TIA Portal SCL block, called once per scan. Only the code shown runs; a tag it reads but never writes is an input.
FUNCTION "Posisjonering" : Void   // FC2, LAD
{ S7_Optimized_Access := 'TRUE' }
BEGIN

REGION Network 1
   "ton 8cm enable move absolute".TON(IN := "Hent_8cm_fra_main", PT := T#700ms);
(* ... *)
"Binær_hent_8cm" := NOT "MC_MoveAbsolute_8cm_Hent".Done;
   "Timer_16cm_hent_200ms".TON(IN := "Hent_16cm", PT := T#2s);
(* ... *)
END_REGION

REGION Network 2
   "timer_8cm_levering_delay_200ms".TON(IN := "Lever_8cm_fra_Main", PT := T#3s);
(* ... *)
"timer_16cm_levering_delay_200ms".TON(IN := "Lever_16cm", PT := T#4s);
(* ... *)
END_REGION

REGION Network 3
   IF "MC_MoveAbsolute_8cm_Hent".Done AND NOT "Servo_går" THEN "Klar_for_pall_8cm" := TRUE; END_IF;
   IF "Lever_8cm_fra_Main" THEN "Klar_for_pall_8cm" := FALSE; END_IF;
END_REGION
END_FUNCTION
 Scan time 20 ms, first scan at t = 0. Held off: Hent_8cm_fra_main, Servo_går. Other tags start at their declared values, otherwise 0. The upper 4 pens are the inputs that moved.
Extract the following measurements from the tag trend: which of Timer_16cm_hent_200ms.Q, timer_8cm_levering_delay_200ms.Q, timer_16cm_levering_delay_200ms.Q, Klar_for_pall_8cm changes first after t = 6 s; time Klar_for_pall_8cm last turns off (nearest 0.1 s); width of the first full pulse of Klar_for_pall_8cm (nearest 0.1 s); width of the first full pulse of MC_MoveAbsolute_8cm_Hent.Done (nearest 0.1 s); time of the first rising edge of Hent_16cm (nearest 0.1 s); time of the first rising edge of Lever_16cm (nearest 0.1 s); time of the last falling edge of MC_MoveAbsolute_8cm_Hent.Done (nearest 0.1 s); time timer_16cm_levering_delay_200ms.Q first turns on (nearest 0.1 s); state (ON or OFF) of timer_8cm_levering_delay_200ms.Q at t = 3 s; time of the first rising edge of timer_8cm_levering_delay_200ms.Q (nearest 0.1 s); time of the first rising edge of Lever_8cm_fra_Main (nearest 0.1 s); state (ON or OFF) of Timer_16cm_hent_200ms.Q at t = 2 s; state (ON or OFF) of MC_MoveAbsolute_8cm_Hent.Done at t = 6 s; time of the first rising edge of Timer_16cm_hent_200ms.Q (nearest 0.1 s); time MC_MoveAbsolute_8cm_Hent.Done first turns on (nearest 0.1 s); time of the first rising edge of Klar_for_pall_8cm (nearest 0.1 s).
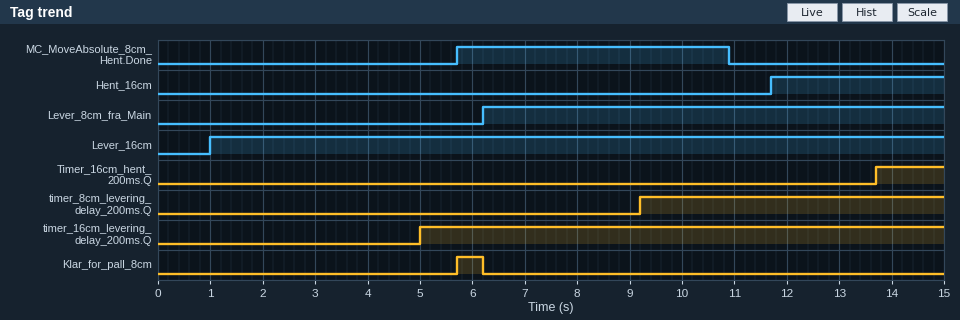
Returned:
Klar_for_pall_8cm
6.2 s
0.5 s
5.2 s
11.7 s
1.0 s
10.9 s
5.0 s
OFF
9.2 s
6.2 s
OFF
ON
13.7 s
5.7 s
5.7 s
